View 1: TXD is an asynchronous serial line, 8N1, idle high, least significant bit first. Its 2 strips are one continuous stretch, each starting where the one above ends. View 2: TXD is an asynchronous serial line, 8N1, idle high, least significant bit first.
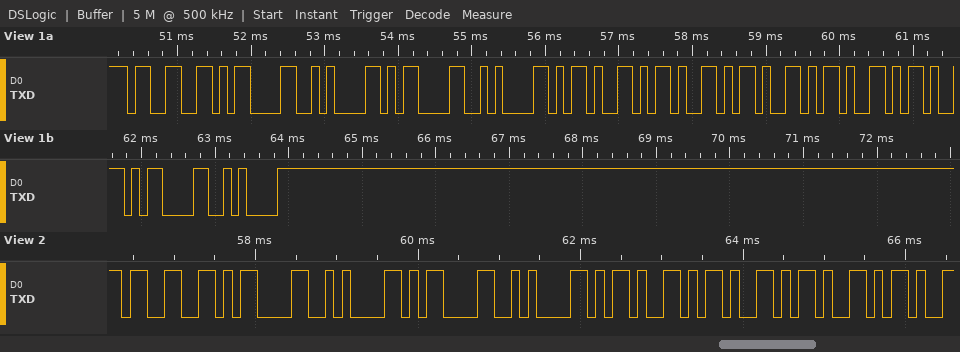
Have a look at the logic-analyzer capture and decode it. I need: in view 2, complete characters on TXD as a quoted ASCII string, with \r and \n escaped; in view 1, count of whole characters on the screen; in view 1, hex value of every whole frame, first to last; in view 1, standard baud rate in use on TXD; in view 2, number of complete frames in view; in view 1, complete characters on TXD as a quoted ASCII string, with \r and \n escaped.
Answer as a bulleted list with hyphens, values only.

- "3\r\n\r\n----"
- 12
- 33 0D 0A 0D 0A 2D 2D 2D 2D 2D 0D 0A
- 9600 baud
- 9
- "3\r\n\r\n-----\r\n"
